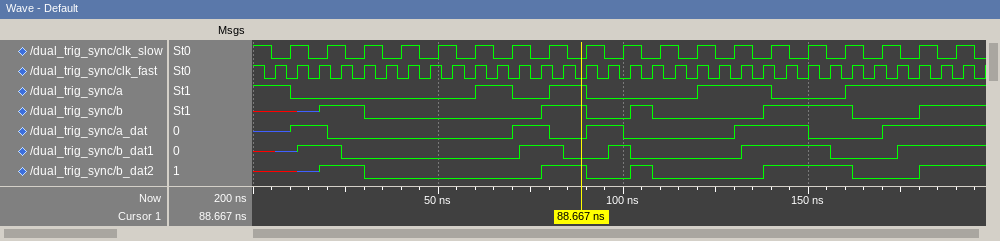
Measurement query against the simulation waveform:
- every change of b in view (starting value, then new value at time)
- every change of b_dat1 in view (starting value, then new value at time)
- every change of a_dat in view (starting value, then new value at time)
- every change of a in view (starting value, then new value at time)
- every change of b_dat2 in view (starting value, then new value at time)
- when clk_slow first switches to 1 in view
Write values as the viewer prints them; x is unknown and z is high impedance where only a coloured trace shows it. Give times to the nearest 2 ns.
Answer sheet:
x, z at 12 ns, 1 at 18 ns, 0 at 30 ns, 1 at 78 ns, 0 at 90 ns, 1 at 102 ns, 0 at 108 ns, 1 at 138 ns, 0 at 162 ns, 1 at 180 ns
x, z at 6 ns, 1 at 12 ns, 0 at 24 ns, 1 at 72 ns, 0 at 84 ns, 1 at 96 ns, 0 at 102 ns, 1 at 132 ns, 0 at 156 ns, 1 at 174 ns
z, 1 at 10 ns, 0 at 20 ns, 1 at 70 ns, 0 at 80 ns, 1 at 90 ns, 0 at 100 ns, 1 at 130 ns, 0 at 150 ns, 1 at 170 ns
1, 0 at 10 ns, 1 at 60 ns, 0 at 70 ns, 1 at 80 ns, 0 at 90 ns, 1 at 120 ns, 0 at 140 ns, 1 at 160 ns
x, z at 12 ns, 1 at 18 ns, 0 at 30 ns, 1 at 78 ns, 0 at 90 ns, 1 at 102 ns, 0 at 108 ns, 1 at 138 ns, 0 at 162 ns, 1 at 180 ns
10 ns
